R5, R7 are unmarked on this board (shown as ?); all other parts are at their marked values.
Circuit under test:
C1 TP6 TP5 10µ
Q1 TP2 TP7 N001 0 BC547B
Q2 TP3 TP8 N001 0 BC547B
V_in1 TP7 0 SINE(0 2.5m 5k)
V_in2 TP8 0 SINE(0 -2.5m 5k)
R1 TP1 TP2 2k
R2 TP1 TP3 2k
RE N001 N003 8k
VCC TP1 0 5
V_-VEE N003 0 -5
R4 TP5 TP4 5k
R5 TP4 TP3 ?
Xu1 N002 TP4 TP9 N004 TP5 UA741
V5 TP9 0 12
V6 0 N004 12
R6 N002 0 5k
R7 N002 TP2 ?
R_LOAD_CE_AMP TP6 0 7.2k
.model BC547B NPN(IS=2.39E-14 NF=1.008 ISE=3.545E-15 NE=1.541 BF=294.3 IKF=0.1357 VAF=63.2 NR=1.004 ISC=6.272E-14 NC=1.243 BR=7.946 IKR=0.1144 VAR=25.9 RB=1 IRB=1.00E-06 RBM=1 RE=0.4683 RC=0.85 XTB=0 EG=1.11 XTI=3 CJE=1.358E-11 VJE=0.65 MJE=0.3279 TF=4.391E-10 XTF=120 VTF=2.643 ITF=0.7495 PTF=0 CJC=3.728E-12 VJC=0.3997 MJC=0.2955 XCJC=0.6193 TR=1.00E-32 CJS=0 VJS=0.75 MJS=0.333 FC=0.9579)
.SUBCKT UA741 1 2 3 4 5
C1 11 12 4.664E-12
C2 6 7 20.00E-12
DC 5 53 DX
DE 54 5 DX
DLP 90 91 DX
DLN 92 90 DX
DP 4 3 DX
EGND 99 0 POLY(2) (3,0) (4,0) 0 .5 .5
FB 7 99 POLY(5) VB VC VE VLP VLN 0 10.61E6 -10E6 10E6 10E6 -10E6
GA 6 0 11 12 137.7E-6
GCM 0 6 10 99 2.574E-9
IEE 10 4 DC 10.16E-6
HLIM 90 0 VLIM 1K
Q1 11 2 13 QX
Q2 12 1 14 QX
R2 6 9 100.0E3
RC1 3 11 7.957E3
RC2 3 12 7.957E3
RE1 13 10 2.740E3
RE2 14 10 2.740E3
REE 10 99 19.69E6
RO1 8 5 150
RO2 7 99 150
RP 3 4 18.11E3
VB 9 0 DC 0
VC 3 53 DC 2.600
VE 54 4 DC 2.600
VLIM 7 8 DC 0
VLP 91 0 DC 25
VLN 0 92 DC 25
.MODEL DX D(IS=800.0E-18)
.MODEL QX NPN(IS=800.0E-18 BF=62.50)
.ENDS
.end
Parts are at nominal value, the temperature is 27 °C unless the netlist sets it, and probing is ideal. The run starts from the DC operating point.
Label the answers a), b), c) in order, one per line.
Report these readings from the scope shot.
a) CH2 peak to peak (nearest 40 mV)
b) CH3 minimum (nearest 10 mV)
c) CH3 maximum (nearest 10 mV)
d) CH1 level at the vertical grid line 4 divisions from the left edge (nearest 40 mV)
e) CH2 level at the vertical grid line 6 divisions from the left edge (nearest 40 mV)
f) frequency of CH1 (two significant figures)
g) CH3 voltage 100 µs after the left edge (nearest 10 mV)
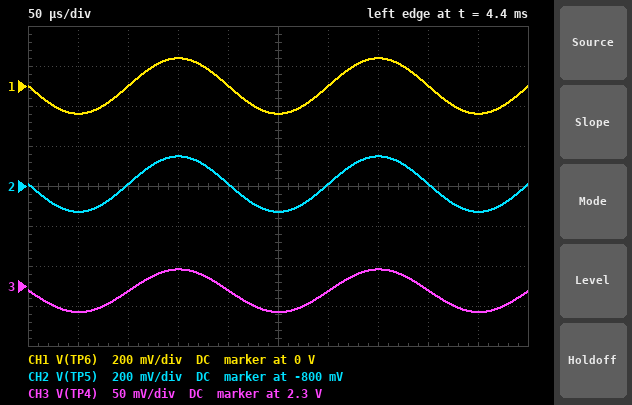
a) 280 mV
b) 2.27 V
c) 2.32 V
d) 0 V
e) -800 mV
f) 5.0 kHz
g) 2.29 V
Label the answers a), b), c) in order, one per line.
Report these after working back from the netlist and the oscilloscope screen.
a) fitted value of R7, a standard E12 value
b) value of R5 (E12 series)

a) 2.7 kΩ
b) 1.5 kΩ
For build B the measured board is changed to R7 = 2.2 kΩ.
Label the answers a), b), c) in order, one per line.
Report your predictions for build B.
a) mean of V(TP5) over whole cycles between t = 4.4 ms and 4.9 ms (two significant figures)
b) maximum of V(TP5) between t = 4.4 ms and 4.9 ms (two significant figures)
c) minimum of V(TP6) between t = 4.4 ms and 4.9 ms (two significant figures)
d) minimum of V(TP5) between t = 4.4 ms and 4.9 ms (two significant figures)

a) -490 mV
b) -340 mV
c) -140 mV
d) -630 mV
